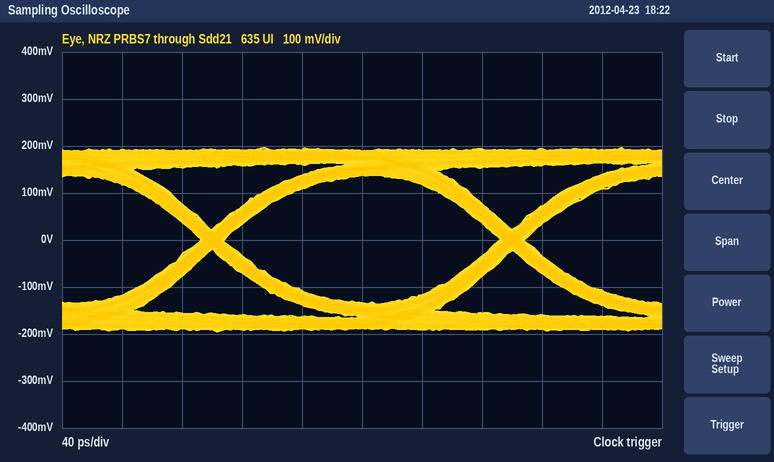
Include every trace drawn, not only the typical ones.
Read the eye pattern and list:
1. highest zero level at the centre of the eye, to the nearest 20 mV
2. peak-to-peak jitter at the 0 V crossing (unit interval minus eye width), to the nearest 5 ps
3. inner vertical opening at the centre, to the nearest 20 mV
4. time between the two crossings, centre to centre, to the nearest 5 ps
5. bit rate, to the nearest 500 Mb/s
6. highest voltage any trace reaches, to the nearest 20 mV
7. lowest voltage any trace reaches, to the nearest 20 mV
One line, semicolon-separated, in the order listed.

-140 mV; 15 ps; 280 mV; 200 ps; 5.0 Gb/s; 200 mV; -200 mV
